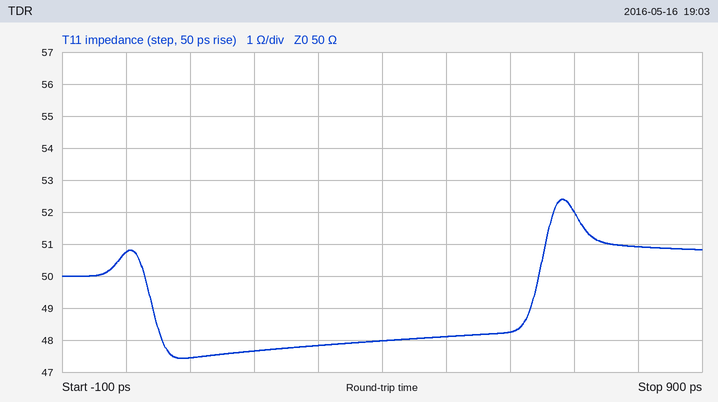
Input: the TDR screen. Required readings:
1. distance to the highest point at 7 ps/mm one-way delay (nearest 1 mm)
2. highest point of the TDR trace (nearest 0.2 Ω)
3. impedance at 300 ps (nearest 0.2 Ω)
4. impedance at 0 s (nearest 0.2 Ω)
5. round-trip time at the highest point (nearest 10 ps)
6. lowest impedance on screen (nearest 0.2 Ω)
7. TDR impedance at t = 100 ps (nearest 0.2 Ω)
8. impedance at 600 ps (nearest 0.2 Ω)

49 mm
52.4 Ω
47.8 Ω
50.8 Ω
680 ps
47.4 Ω
47.4 Ω
48.2 Ω
